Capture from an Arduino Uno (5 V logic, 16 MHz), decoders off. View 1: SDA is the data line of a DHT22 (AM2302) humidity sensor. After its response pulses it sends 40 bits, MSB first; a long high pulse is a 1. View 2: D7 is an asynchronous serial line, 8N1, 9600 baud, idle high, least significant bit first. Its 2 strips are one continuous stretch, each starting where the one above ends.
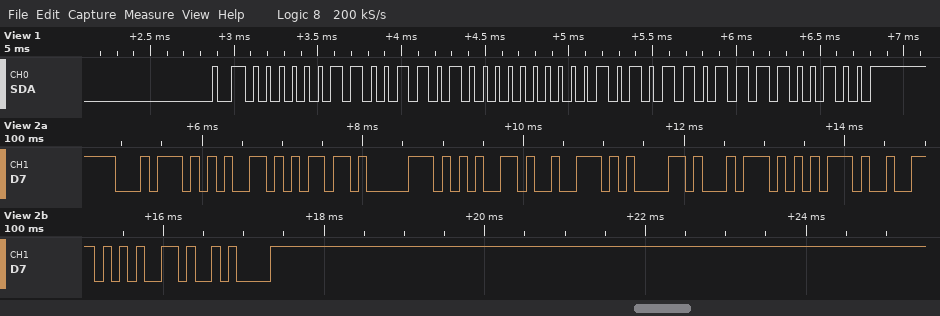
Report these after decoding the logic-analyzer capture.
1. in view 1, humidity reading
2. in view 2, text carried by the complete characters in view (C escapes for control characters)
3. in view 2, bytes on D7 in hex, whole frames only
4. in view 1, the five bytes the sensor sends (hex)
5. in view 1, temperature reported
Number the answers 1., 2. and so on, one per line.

1. 82.0 %
2. "temperature\n"
3. 74 65 6D 70 65 72 61 74 75 72 65 0A
4. 03 34 00 AD E4
5. 17.3 °C
